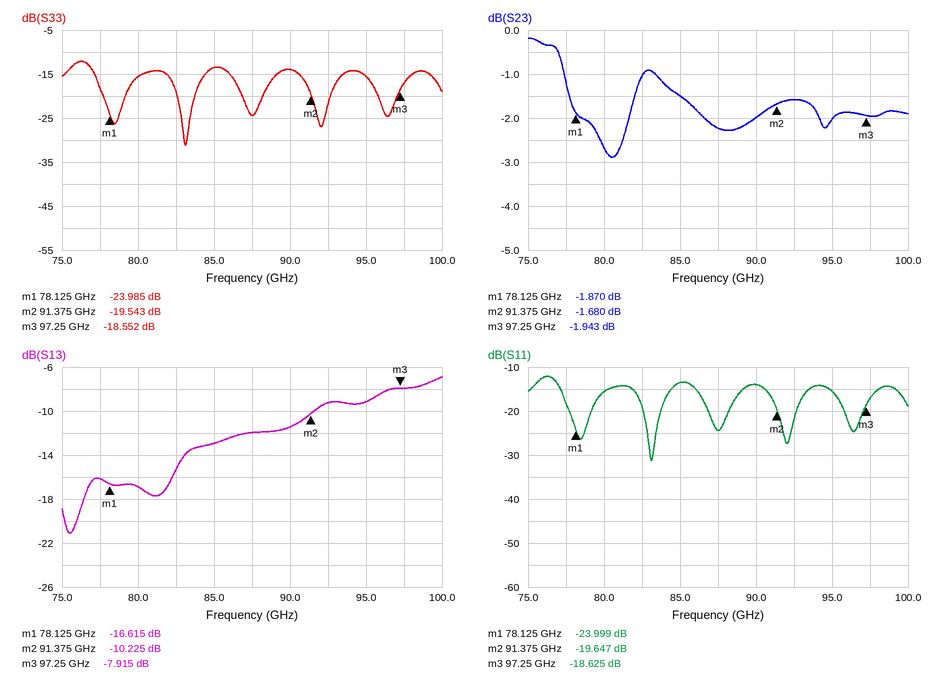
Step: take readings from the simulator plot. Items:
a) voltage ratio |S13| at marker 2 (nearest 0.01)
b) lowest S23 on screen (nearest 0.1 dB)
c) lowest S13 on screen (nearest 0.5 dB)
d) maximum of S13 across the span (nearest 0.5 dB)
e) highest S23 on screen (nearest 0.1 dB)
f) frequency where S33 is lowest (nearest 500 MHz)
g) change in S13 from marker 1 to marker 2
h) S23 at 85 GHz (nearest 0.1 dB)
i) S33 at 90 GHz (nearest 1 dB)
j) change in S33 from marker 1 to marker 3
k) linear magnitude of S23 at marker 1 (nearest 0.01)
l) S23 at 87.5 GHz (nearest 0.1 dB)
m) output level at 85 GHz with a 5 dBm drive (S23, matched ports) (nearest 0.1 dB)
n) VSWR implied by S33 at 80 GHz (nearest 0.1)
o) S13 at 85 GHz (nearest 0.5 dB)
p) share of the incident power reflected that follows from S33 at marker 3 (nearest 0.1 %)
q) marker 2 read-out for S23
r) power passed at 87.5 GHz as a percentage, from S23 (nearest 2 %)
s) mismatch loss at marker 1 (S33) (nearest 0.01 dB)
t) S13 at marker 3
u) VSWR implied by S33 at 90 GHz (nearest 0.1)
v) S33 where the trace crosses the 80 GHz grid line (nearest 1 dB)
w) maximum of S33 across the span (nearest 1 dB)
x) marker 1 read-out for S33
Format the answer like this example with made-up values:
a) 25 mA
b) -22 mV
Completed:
a) 0.31
b) -2.9 dB
c) -21.0 dB
d) -7.0 dB
e) -0.2 dB
f) 83.0 GHz
g) 6.390 dB
h) -1.5 dB
i) -14 dB
j) 5.433 dB
k) 0.81
l) -2.2 dB
m) 3.5 dBm
n) 1.4
o) -13.0 dB
p) 1.4 %
q) -1.680 dB
r) 60 %
s) 0.02 dB
t) -7.915 dB
u) 1.5
v) -16 dB
w) -12 dB
x) -23.985 dB
